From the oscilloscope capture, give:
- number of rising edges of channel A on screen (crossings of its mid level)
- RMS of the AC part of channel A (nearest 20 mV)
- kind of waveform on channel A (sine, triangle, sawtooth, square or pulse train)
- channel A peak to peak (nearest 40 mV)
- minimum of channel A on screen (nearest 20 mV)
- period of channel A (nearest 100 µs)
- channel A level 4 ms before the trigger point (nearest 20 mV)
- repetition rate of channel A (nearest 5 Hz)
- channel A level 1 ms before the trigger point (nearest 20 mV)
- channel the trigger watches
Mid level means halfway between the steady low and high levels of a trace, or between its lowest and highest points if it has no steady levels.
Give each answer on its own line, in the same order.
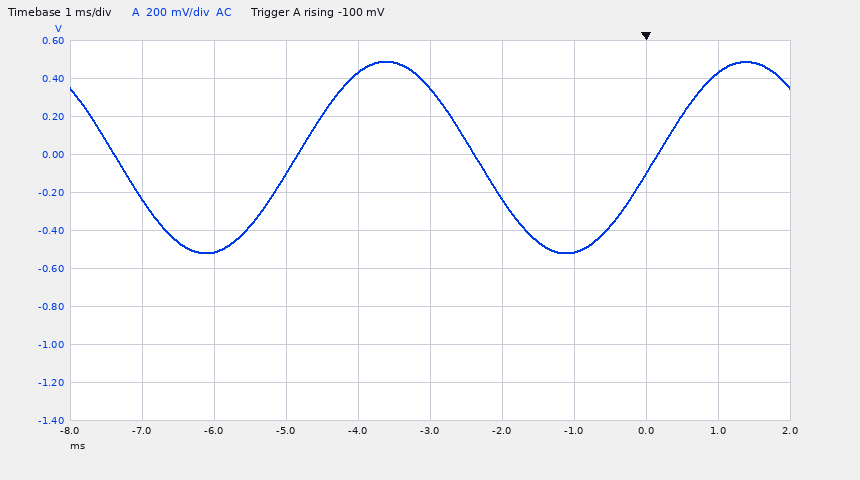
2
360 mV
sine
1.00 V
-520 mV
5.0 ms
440 mV
200 Hz
-520 mV
channel A
